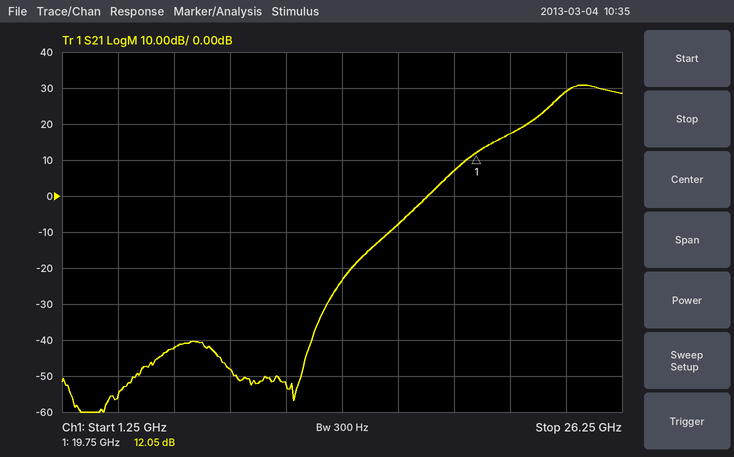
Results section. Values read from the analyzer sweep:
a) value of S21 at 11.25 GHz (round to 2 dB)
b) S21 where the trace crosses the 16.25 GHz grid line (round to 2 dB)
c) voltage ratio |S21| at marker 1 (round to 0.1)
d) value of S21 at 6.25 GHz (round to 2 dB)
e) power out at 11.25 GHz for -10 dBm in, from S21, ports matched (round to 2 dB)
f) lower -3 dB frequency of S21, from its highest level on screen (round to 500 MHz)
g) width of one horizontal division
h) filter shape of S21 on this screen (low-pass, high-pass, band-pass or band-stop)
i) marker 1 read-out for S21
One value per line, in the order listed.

-52 dB
-8 dB
4.0
-42 dB
-62 dBm
23.5 GHz
2.5 GHz
high-pass
12.05 dB
